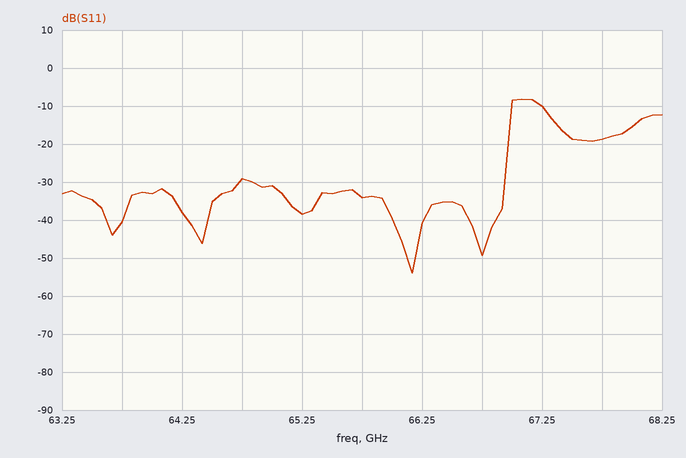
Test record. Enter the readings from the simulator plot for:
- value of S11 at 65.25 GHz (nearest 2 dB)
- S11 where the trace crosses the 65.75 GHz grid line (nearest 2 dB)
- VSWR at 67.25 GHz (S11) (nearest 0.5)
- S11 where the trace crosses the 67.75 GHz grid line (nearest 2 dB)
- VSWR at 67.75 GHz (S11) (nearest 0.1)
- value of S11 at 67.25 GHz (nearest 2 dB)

-38 dB
-34 dB
2.0
-18 dB
1.3
-10 dB
